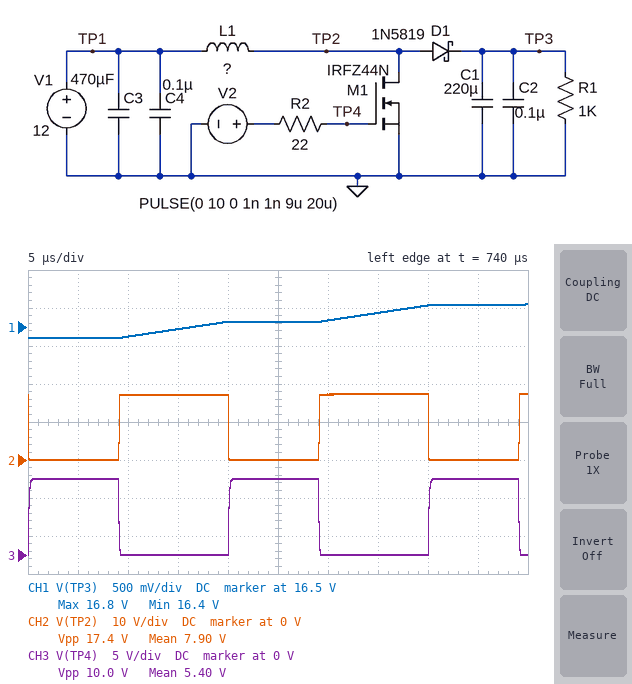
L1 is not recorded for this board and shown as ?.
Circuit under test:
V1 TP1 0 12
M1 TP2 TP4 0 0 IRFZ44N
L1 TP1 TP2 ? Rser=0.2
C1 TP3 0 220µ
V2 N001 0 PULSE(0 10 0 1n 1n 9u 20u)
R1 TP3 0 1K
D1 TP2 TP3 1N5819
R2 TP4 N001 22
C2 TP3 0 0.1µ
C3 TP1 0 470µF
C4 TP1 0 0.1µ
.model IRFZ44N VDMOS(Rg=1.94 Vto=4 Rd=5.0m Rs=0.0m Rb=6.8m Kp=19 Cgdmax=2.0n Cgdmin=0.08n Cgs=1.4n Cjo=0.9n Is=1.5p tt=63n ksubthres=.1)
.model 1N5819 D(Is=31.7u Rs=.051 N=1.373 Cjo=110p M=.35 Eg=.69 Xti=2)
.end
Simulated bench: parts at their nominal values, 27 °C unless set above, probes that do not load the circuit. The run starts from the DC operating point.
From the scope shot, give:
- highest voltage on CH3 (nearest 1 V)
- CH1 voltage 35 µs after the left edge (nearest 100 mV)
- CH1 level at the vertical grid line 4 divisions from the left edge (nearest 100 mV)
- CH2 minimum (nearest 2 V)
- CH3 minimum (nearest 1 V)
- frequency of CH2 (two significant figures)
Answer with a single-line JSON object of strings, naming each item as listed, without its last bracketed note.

{"highest voltage on CH3": "10 V", "CH1 voltage 35 µs after the left edge": "16.7 V", "CH1 level at the vertical grid line 4 divisions from the left edge": "16.6 V", "CH2 minimum": "0 V", "CH3 minimum": "0 V", "frequency of CH2": "50 kHz"}
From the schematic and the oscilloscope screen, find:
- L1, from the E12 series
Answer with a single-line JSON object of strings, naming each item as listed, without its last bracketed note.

{"L1, from the E12 series": "680 µH"}
